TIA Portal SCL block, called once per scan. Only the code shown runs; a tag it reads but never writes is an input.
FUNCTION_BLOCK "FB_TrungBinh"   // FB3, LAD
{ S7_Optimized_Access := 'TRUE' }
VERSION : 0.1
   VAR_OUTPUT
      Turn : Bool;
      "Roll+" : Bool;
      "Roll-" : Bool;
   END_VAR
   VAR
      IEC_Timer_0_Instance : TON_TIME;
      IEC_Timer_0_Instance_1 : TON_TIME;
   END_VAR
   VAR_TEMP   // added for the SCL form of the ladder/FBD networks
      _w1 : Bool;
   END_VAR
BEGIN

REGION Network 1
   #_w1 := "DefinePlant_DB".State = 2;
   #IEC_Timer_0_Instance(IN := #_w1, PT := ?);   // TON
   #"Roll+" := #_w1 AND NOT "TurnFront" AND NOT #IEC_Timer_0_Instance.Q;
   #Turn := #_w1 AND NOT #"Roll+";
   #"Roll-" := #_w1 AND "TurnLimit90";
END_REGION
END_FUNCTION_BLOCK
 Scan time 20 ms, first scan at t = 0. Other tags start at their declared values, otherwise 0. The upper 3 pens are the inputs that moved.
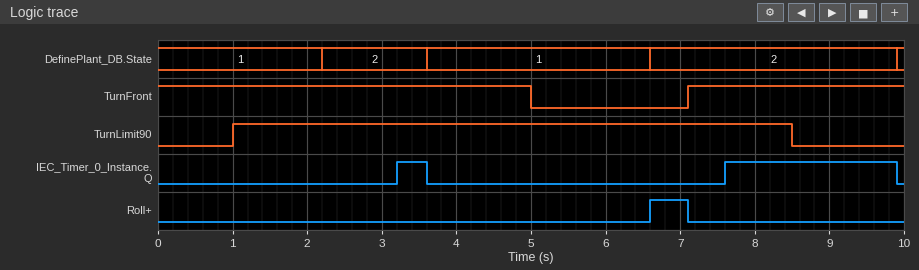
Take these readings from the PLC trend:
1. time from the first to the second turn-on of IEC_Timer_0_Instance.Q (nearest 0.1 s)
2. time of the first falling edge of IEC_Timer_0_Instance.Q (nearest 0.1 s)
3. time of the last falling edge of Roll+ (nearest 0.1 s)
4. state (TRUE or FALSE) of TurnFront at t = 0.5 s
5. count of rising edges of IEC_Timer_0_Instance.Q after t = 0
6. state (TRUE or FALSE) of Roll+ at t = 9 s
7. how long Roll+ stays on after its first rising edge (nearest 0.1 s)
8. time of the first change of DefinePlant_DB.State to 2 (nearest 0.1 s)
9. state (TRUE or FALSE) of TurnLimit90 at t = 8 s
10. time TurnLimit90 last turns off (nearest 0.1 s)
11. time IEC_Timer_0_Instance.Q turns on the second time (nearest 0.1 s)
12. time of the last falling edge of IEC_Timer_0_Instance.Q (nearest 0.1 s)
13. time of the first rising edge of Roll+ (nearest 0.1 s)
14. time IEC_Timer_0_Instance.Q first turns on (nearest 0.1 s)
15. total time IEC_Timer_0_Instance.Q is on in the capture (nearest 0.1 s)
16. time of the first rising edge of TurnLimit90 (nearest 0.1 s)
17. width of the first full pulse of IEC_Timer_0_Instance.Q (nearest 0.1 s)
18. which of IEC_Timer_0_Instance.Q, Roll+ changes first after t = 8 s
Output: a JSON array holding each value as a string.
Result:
["4.4 s", "3.6 s", "7.1 s", "TRUE", "2", "FALSE", "0.5 s", "2.2 s", "TRUE", "8.5 s", "7.6 s", "9.9 s", "6.6 s", "3.2 s", "2.7 s", "1.0 s", "0.4 s", "IEC_Timer_0_Instance.Q"]
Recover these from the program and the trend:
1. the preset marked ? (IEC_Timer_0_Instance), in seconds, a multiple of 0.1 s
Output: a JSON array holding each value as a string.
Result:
["1.0 s"]
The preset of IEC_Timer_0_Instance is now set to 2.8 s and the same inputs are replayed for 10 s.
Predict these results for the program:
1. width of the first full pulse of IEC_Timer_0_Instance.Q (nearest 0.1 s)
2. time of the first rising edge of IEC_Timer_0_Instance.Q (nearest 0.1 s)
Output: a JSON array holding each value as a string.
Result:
["0.5 s", "9.4 s"]
